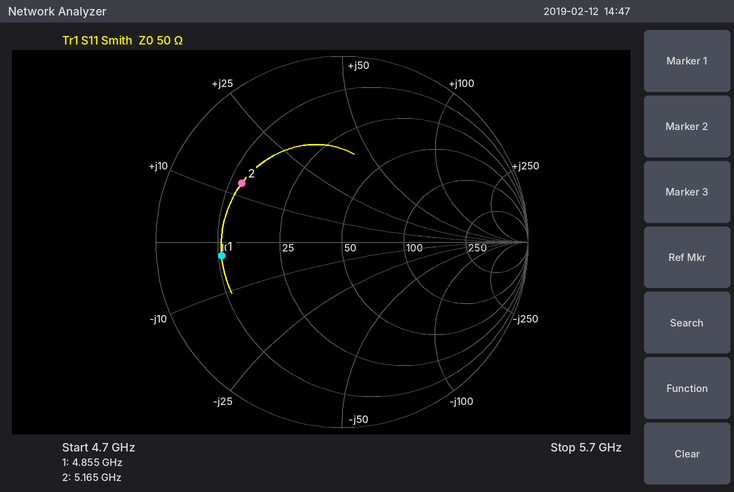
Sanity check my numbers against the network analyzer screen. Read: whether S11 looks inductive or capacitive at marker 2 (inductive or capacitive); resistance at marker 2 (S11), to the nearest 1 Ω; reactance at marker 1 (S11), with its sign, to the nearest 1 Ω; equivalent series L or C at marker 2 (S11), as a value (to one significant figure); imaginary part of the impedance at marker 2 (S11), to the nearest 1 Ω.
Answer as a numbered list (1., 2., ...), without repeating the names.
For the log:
1. inductive
2. 12 Ω
3. -3 Ω
4. 400 pH
5. +13 Ω
